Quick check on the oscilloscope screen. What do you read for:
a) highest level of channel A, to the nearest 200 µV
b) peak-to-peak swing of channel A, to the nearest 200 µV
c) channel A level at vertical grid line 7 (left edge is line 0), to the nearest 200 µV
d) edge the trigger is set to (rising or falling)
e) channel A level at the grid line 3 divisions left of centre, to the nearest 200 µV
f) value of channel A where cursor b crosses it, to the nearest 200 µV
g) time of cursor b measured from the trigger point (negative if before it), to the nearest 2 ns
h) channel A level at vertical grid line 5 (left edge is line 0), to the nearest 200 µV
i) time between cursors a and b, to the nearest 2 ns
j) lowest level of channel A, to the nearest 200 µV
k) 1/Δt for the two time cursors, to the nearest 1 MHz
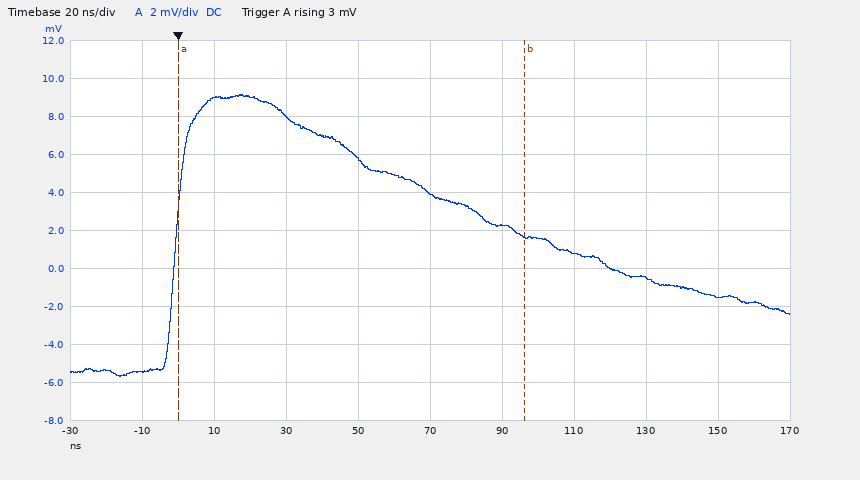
9.2 mV
14.8 mV
800 µV
rising
9.0 mV
1.6 mV
+96 ns
4.0 mV
96 ns
-5.6 mV
10 MHz
